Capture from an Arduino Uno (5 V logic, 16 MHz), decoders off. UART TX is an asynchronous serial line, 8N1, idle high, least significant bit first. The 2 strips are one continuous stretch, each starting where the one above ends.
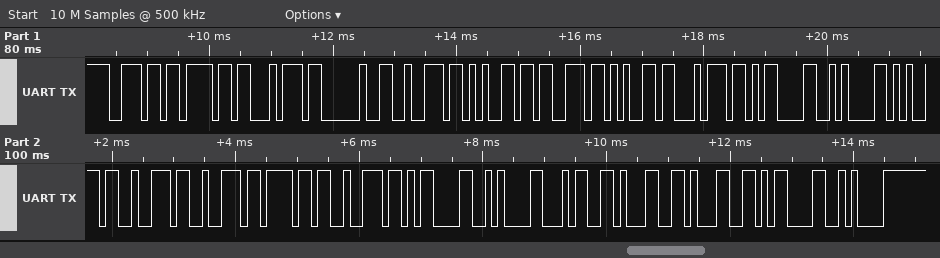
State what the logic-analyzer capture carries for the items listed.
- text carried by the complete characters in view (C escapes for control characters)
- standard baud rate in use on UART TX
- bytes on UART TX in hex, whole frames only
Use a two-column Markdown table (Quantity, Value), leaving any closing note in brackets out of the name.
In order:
| Quantity | Value |
|---|---|
| text carried by the complete characters in view | "not reset\r\nerror\r\n411\r\n" |
| standard baud rate in use on UART TX | 9600 baud |
| bytes on UART TX in hex, whole frames only | 6E 6F 74 20 72 65 73 65 74 0D 0A 65 72 72 6F 72 0D 0A 34 31 31 0D 0A |
